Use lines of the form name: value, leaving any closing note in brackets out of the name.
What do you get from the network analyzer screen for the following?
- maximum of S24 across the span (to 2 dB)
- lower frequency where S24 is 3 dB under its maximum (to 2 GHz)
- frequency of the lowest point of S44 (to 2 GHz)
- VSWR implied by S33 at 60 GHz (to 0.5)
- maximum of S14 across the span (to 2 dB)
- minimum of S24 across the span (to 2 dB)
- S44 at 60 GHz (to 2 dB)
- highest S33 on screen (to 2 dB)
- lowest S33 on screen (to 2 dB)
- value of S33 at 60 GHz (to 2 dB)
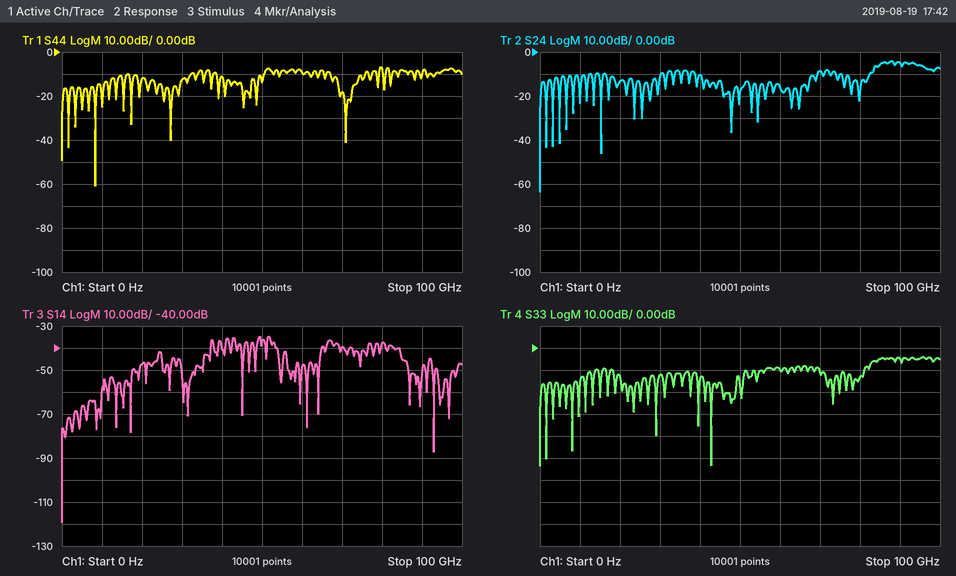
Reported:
maximum of S24 across the span: -4 dB
lower frequency where S24 is 3 dB under its maximum: 84 GHz
frequency of the lowest point of S44: 8 GHz
VSWR implied by S33 at 60 GHz: 2.0
maximum of S14 across the span: -34 dB
minimum of S24 across the span: -64 dB
S44 at 60 GHz: -10 dB
highest S33 on screen: -4 dB
lowest S33 on screen: -54 dB
value of S33 at 60 GHz: -10 dB
